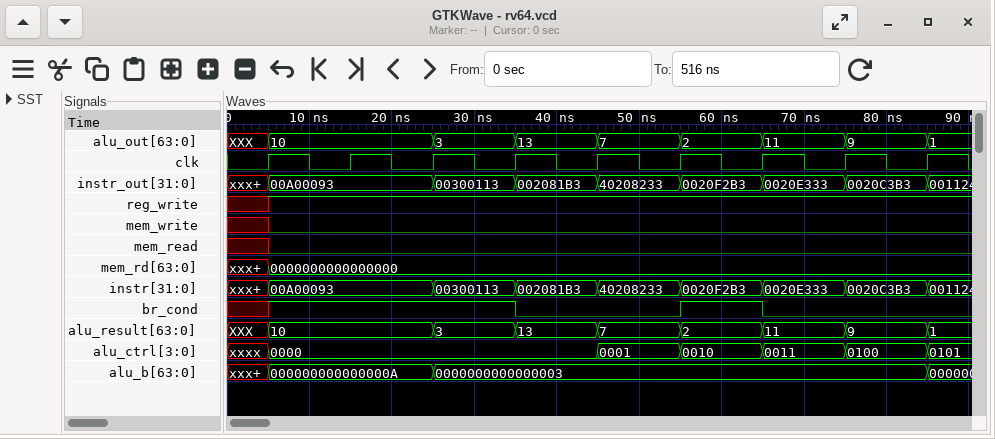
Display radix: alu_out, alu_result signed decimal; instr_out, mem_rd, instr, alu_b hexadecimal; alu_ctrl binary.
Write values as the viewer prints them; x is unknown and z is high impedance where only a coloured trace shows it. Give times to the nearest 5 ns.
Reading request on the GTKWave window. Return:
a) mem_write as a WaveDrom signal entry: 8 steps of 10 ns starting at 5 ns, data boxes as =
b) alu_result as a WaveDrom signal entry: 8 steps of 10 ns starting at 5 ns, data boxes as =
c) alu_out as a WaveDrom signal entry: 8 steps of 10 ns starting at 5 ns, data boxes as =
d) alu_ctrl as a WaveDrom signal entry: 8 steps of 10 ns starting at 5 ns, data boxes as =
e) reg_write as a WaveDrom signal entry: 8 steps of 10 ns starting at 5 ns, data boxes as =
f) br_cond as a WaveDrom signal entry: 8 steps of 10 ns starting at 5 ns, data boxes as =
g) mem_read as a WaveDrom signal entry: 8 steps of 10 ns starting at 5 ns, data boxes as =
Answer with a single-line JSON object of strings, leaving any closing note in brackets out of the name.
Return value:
{"mem_write as a WaveDrom signal entry: 8 steps of 10 ns starting at 5 ns, data boxes as =": "{name: 'mem_write', wave: '0.......'}", "alu_result as a WaveDrom signal entry: 8 steps of 10 ns starting at 5 ns, data boxes as =": "{name: 'alu_result', wave: '=.======', data: '10 3 13 7 2 11 9'}", "alu_out as a WaveDrom signal entry: 8 steps of 10 ns starting at 5 ns, data boxes as =": "{name: 'alu_out', wave: '=.======', data: '10 3 13 7 2 11 9'}", "alu_ctrl as a WaveDrom signal entry: 8 steps of 10 ns starting at 5 ns, data boxes as =": "{name: 'alu_ctrl', wave: '=...====', data: '0000 0001 0010 0011 0100'}", "reg_write as a WaveDrom signal entry: 8 steps of 10 ns starting at 5 ns, data boxes as =": "{name: 'reg_write', wave: '1.......'}", "br_cond as a WaveDrom signal entry: 8 steps of 10 ns starting at 5 ns, data boxes as =": "{name: 'br_cond', wave: '1..0.10.'}", "mem_read as a WaveDrom signal entry: 8 steps of 10 ns starting at 5 ns, data boxes as =": "{name: 'mem_read', wave: '0.......'}"}
